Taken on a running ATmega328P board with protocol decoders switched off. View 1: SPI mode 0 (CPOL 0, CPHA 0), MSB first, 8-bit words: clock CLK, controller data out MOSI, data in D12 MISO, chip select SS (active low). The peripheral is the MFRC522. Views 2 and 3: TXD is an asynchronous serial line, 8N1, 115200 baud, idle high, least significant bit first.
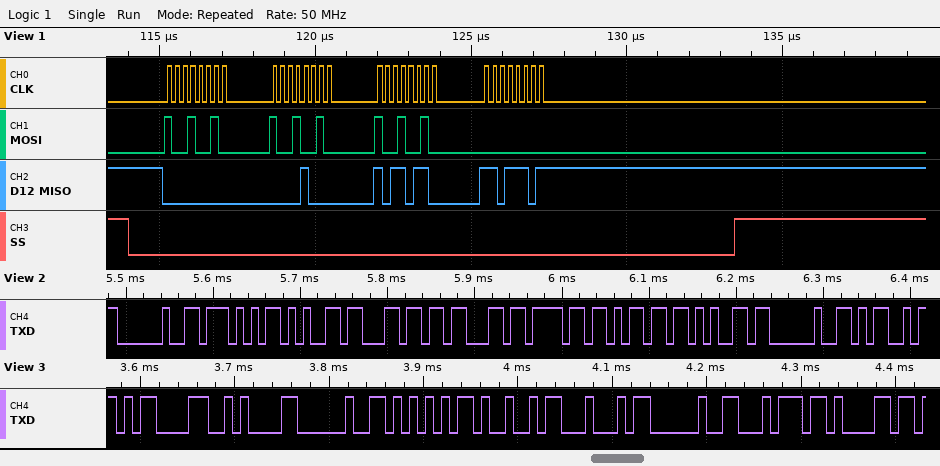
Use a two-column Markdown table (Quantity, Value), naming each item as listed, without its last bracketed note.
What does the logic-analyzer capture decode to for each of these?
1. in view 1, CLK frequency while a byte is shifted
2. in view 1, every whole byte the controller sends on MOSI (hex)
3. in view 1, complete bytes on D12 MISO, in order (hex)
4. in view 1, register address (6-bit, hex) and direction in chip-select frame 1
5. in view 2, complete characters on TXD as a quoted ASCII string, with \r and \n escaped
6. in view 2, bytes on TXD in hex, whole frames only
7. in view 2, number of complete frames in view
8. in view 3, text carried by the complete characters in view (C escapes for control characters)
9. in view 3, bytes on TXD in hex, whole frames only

| Quantity | Value |
|---|---|
| in view 1, CLK frequency while a byte is shifted | 4 MHz |
| in view 1, every whole byte the controller sends on MOSI | 92 92 92 00 |
| in view 1, complete bytes on D12 MISO, in order | 00 08 B6 DD |
| in view 1, register address (6-bit, hex) and direction in chip-select frame 1 | 0x09 read |
| in view 2, complete characters on TXD as a quoted ASCII string, with \r and \n escaped | " Welcome M" |
| in view 2, bytes on TXD in hex, whole frames only | 20 57 65 6C 63 6F 6D 65 20 4D |
| in view 2, number of complete frames in view | 10 |
| in view 3, text carried by the complete characters in view | "\r\n UID ta" |
| in view 3, bytes on TXD in hex, whole frames only | 0D 0A 20 55 49 44 20 74 61 |
